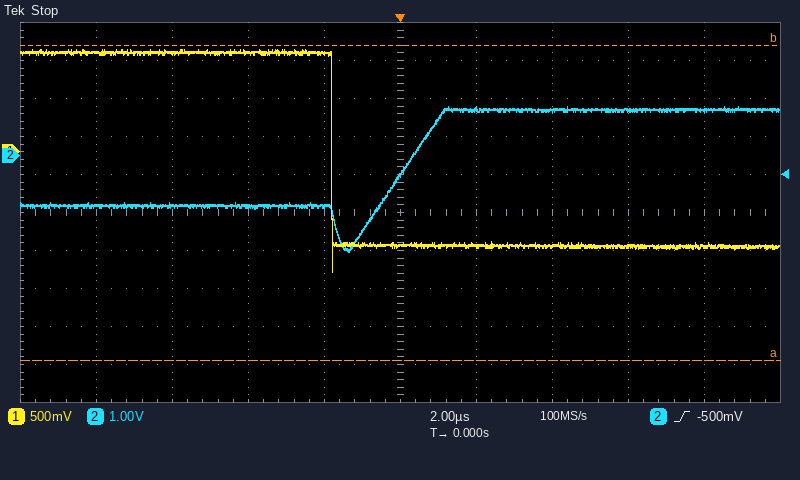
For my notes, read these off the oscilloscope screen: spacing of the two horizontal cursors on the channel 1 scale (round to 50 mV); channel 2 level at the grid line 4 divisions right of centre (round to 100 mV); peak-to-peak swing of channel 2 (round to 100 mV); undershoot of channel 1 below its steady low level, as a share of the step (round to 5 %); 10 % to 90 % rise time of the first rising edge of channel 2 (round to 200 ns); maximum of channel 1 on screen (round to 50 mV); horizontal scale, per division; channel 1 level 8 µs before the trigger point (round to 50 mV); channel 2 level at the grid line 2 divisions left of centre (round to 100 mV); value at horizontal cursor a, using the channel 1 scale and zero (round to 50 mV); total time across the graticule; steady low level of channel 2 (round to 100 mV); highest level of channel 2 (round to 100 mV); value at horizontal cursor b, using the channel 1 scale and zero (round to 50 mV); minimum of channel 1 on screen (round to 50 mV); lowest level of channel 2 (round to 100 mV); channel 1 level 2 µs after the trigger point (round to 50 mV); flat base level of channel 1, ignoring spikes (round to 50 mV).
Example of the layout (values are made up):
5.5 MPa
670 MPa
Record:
4.15 V
1.2 V
3.8 V
15 %
1.4 µs
1.35 V
2 µs
1.30 V
-1.3 V
-2.75 V
20 µs
-1.3 V
1.3 V
1.40 V
-1.60 V
-2.5 V
-1.25 V
-1.25 V
